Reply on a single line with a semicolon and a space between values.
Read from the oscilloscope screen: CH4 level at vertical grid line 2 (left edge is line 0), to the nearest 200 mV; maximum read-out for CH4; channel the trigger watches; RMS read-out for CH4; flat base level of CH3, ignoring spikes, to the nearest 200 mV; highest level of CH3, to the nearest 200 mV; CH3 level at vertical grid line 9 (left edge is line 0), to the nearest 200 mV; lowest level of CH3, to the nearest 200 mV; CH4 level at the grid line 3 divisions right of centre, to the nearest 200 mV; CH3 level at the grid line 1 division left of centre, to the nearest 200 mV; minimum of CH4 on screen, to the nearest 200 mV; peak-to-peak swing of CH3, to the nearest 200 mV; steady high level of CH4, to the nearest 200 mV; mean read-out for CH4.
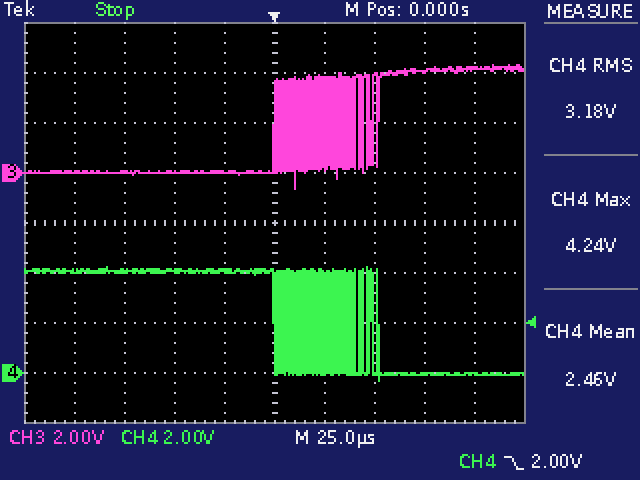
4.0 V; 4.24 V; CH4; 3.18 V; 0.0 V; 4.4 V; 4.2 V; -600 mV; 0.0 V; 0.0 V; -400 mV; 5.0 V; 4.0 V; 2.46 V
